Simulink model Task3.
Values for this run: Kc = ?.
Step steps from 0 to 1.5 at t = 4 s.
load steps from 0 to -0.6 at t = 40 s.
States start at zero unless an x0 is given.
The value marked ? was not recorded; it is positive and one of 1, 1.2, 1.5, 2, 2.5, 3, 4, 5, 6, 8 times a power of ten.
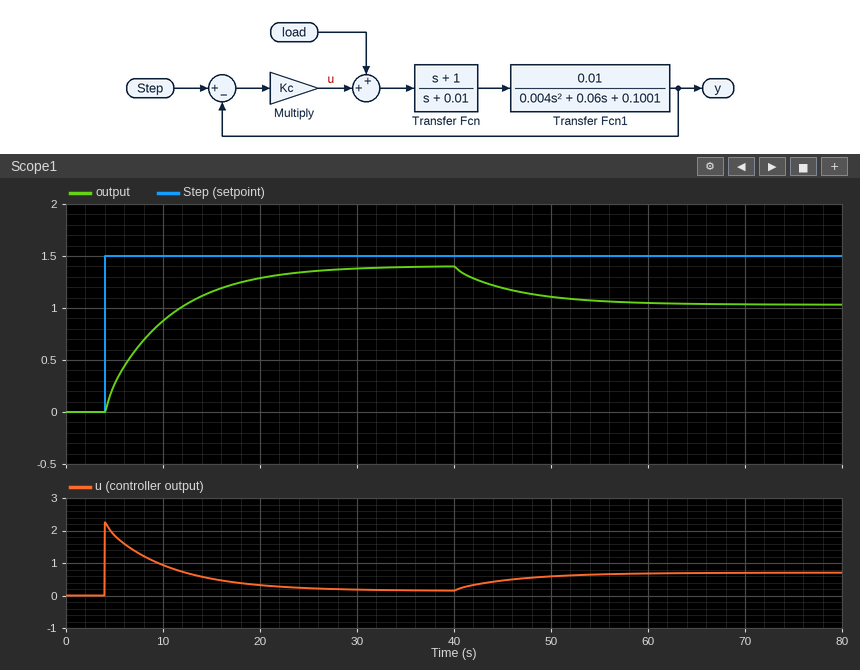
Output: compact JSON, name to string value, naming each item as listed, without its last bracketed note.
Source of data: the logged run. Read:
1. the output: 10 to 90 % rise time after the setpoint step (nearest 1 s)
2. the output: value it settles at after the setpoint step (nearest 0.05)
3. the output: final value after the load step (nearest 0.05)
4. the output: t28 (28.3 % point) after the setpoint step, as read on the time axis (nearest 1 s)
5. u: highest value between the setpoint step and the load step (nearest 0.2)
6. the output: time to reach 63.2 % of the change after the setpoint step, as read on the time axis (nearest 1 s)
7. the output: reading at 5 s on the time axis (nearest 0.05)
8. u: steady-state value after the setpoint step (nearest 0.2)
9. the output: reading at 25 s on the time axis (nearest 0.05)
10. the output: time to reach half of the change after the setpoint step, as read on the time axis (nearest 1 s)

{"the output: 10 to 90 % rise time after the setpoint step": "14 s", "the output: value it settles at after the setpoint step": "1.40", "the output: final value after the load step": "1.05", "the output: t28 (28.3 % point) after the setpoint step, as read on the time axis": "6 s", "u: highest value between the setpoint step and the load step": "2.2", "the output: time to reach 63.2 % of the change after the setpoint step, as read on the time axis": "10 s", "the output: reading at 5 s on the time axis": "0.25", "u: steady-state value after the setpoint step": "0.2", "the output: reading at 25 s on the time axis": "1.35", "the output: time to reach half of the change after the setpoint step, as read on the time axis": "8 s"}
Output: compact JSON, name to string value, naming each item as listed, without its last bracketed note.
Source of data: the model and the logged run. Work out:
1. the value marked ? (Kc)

{"the value marked ?": "1.5"}
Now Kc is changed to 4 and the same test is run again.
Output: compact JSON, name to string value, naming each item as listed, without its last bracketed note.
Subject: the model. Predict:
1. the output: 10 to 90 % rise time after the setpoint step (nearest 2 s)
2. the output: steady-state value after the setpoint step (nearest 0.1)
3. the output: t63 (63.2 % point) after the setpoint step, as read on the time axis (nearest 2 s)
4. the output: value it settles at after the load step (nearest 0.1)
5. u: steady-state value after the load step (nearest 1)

{"the output: 10 to 90 % rise time after the setpoint step": "6 s", "the output: steady-state value after the setpoint step": "1.5", "the output: t63 (63.2 % point) after the setpoint step, as read on the time axis": "6 s", "the output: value it settles at after the load step": "1.3", "u: steady-state value after the load step": "1"}
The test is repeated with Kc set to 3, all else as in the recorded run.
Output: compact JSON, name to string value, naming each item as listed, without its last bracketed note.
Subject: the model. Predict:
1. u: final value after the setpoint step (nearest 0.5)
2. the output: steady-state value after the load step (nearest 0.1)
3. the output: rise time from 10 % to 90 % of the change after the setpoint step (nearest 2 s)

{"u: final value after the setpoint step": "0.0", "the output: steady-state value after the load step": "1.3", "the output: rise time from 10 % to 90 % of the change after the setpoint step": "8 s"}
